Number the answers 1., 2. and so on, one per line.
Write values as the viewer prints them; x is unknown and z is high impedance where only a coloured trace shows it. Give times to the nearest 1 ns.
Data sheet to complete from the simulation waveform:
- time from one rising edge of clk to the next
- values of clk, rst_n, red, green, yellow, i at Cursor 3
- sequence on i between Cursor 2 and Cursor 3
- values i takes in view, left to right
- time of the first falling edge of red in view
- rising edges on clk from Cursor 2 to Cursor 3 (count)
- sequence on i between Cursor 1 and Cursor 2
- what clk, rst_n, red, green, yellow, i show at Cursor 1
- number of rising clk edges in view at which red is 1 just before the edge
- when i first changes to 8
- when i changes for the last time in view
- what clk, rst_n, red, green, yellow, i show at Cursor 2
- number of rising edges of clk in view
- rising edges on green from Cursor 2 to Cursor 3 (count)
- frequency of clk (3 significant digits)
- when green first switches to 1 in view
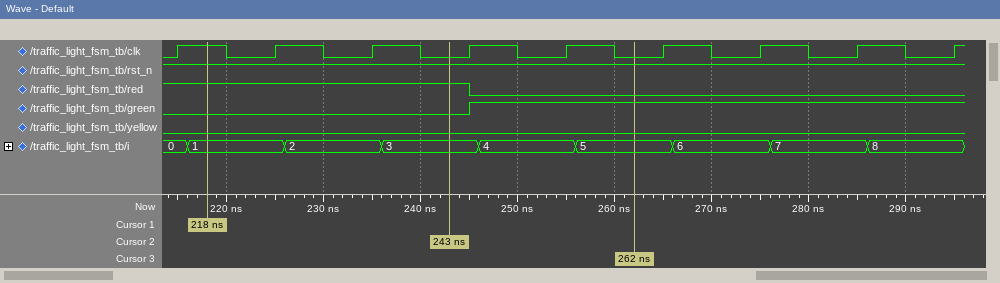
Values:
1. 10 ns
2. clk=0, rst_n=1, red=0, green=1, yellow=0, i=5
3. 3, 4, 5
4. 0, 1, 2, 3, 4, 5, 6, 7, 8
5. 245 ns
6. 2
7. 1, 2, 3
8. clk=1, rst_n=1, red=1, green=0, yellow=0, i=1
9. 4
10. 286 ns
11. 286 ns
12. clk=0, rst_n=1, red=1, green=0, yellow=0, i=3
13. 9
14. 1
15. 100 MHz
16. 245 ns
